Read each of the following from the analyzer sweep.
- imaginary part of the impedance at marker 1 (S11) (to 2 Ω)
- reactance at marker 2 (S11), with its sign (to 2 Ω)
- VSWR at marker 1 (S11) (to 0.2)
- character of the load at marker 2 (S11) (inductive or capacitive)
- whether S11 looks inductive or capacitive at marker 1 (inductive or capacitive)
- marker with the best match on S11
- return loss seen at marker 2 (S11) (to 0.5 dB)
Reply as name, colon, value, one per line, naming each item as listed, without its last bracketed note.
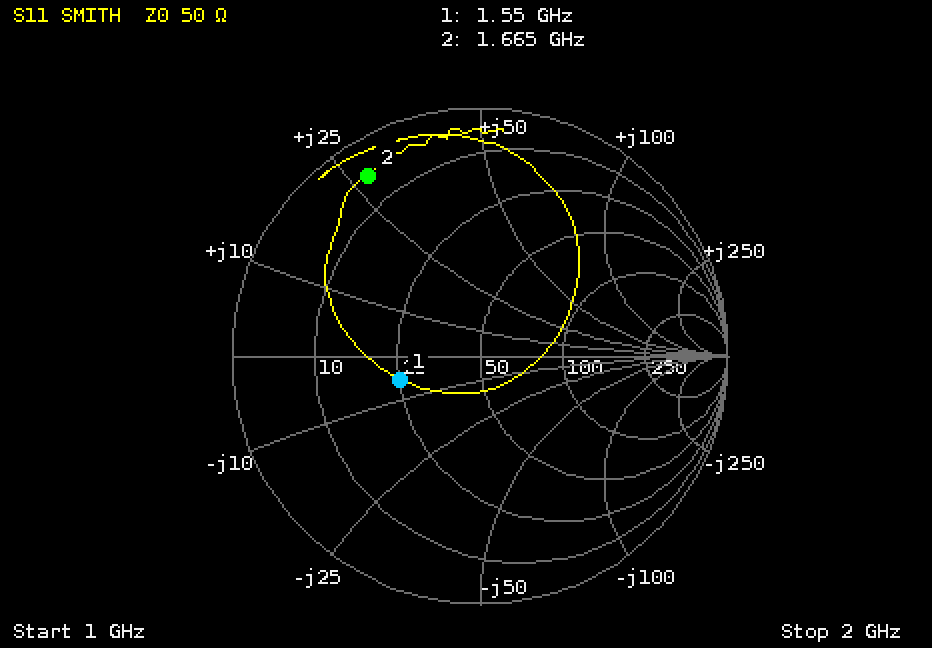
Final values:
imaginary part of the impedance at marker 1 (S11): -6 Ω
reactance at marker 2 (S11), with its sign: +28 Ω
VSWR at marker 1 (S11): 2.0
character of the load at marker 2 (S11): inductive
whether S11 looks inductive or capacitive at marker 1: capacitive
marker with the best match on S11: marker 1
return loss seen at marker 2 (S11): 1.5 dB
